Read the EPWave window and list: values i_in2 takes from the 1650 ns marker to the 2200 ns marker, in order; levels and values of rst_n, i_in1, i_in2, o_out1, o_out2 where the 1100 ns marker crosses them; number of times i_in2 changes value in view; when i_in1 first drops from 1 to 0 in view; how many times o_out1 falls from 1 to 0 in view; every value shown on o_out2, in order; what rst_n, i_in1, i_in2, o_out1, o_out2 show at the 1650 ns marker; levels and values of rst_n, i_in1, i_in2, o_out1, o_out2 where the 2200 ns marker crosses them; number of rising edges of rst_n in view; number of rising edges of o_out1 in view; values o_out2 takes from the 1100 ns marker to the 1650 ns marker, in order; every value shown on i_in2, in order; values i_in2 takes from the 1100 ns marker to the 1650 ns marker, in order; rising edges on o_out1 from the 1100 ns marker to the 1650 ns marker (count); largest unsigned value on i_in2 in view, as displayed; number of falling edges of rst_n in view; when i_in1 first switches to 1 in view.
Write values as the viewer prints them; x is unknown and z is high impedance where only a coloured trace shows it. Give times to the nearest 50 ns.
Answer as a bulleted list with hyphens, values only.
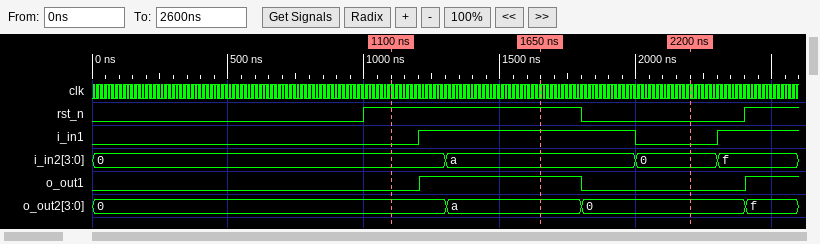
- a, 0
- rst_n=1, i_in1=0, i_in2=0, o_out1=0, o_out2=0
- 3
- 2000 ns
- 1
- 0, a, 0, f
- rst_n=1, i_in1=1, i_in2=a, o_out1=1, o_out2=a
- rst_n=0, i_in1=0, i_in2=0, o_out1=0, o_out2=0
- 2
- 2
- 0, a
- 0, a, 0, f
- 0, a
- 1
- f
- 1
- 1200 ns
